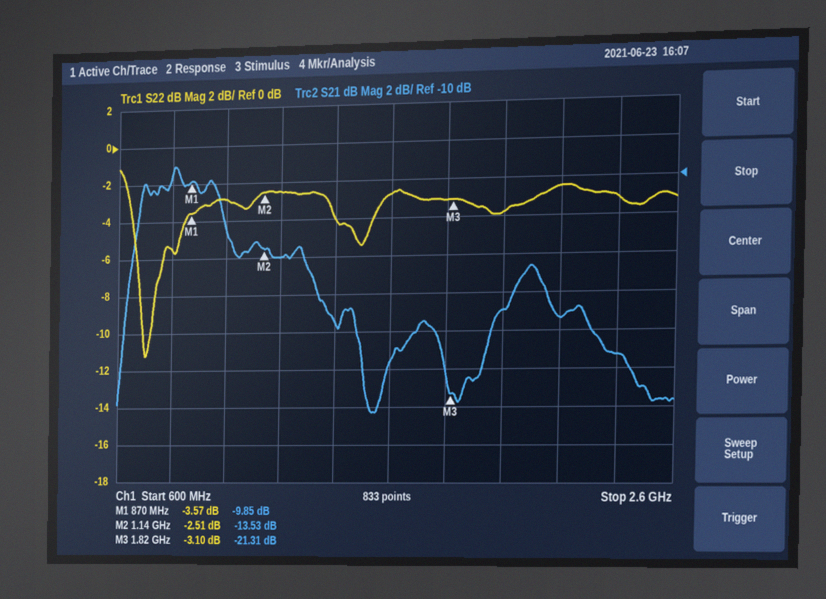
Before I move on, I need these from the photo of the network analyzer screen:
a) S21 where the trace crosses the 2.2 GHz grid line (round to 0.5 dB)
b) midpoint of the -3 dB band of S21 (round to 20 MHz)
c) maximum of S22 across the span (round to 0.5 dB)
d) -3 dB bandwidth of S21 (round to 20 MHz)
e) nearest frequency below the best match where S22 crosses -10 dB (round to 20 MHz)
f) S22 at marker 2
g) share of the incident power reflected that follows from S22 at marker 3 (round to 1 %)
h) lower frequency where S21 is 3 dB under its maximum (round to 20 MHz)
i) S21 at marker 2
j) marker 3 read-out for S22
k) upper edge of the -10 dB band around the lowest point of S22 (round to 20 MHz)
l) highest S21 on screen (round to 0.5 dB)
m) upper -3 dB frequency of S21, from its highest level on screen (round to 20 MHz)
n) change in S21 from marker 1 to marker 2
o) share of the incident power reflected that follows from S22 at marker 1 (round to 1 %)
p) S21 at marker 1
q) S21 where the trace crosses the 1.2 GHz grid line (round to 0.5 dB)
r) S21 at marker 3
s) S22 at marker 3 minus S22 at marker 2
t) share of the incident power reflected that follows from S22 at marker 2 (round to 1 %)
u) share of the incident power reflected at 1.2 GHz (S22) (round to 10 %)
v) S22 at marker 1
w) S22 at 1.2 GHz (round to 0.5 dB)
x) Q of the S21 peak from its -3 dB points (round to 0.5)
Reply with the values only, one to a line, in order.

-17.5 dB
840 MHz
-1.0 dB
320 MHz
700 MHz
-2.51 dB
49 %
680 MHz
-13.53 dB
-3.10 dB
720 MHz
-9.0 dB
1.00 GHz
-3.68 dB
44 %
-9.85 dB
-14.0 dB
-21.31 dB
-0.59 dB
56 %
60 %
-3.57 dB
-2.5 dB
2.5
